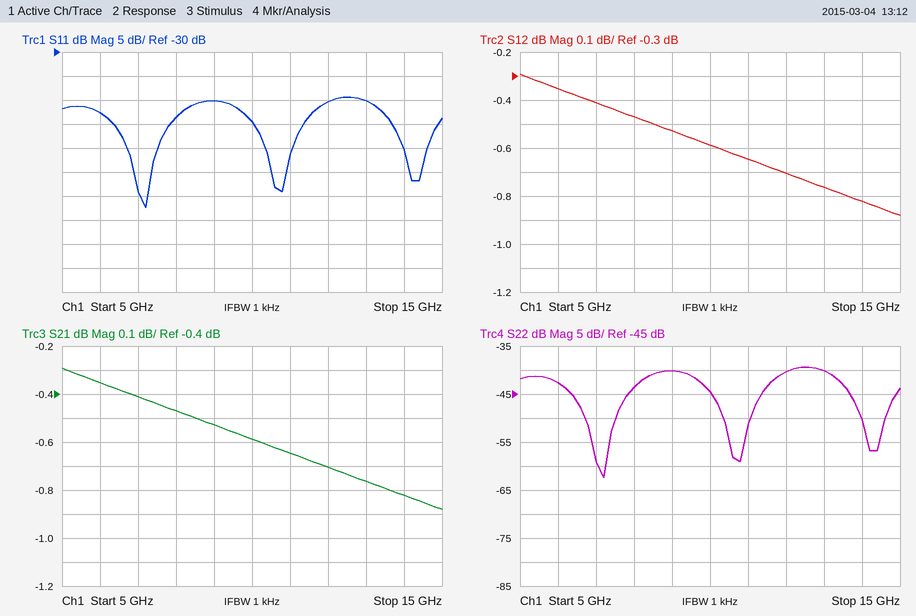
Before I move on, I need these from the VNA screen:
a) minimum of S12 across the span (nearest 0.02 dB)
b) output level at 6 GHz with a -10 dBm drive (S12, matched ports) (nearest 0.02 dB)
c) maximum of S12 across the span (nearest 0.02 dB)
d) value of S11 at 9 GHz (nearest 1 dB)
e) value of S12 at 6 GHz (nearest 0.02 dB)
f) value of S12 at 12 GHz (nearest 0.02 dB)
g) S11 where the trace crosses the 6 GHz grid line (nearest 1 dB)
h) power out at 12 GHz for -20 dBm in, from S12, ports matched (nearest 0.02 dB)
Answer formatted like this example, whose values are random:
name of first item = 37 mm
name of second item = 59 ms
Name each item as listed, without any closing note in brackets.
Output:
minimum of S12 across the span = -0.88 dB
output level at 6 GHz with a -10 dBm drive (S12, matched ports) = -10.36 dBm
maximum of S12 across the span = -0.30 dB
value of S11 at 9 GHz = -40 dB
value of S12 at 6 GHz = -0.36 dB
value of S12 at 12 GHz = -0.70 dB
S11 where the trace crosses the 6 GHz grid line = -43 dB
power out at 12 GHz for -20 dBm in, from S12, ports matched = -20.70 dBm
